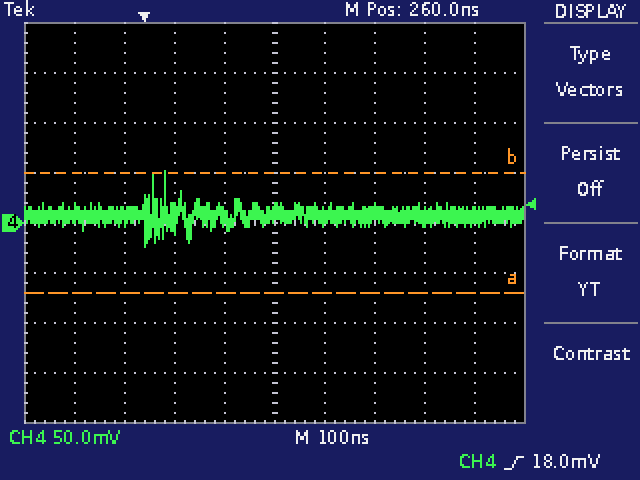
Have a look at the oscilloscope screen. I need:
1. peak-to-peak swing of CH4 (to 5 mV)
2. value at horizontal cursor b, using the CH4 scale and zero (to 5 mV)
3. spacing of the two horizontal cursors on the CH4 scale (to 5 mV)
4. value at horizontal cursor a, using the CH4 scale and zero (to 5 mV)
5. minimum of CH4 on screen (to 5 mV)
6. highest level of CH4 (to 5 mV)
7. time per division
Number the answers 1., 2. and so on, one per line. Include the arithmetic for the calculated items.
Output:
1. 50 mV − (-25 mV) = 75 mV
2. 50 mV
3. 120 mV
4. -70 mV
5. -25 mV
6. 50 mV
7. 100 ns
